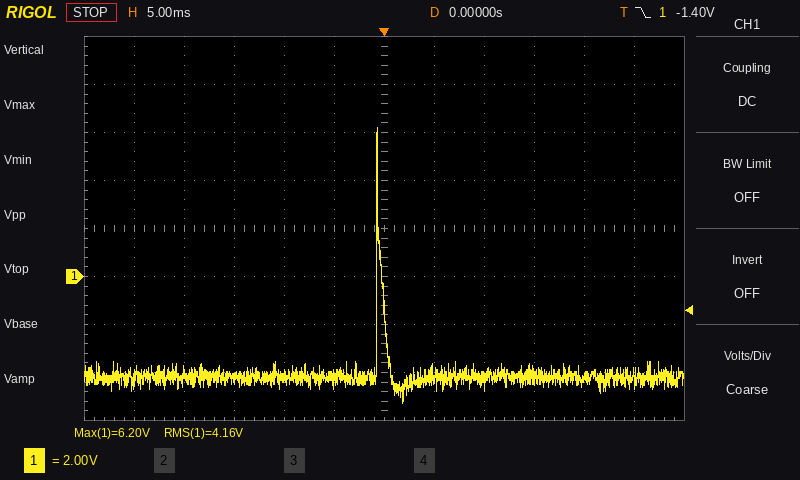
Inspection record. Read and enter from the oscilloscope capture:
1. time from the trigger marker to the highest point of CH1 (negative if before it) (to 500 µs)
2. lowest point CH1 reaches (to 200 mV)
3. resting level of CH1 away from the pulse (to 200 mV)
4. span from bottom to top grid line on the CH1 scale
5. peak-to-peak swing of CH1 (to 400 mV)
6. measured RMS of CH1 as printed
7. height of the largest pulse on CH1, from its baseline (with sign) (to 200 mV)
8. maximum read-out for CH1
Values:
-500 µs
-5.2 V
-4.2 V
16 V
11.6 V
4.16 V
+10.4 V
6.20 V
